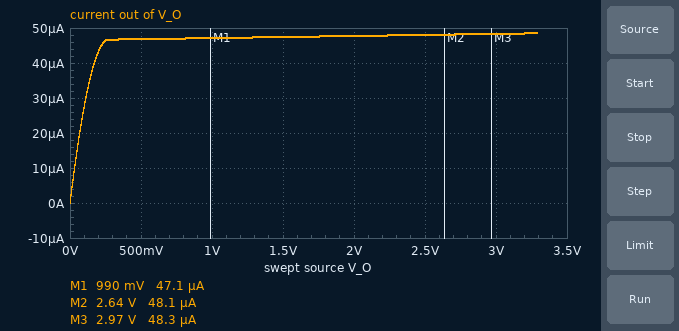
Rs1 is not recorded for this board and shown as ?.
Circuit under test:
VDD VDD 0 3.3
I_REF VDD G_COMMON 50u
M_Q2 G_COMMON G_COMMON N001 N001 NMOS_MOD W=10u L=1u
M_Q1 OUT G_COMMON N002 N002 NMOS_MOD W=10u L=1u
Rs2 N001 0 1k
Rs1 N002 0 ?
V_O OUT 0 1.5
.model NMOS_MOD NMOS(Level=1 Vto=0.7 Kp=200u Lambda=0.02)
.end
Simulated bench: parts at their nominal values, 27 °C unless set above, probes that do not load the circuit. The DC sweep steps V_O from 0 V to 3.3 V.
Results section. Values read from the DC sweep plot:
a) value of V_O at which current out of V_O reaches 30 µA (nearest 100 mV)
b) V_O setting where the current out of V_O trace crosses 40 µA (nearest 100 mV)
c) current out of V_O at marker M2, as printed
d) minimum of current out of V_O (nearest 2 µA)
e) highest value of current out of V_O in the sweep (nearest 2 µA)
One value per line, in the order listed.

100 mV
200 mV
48.1 µA
0 A
48 µA
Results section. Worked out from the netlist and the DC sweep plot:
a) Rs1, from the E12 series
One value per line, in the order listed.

1.2 kΩ
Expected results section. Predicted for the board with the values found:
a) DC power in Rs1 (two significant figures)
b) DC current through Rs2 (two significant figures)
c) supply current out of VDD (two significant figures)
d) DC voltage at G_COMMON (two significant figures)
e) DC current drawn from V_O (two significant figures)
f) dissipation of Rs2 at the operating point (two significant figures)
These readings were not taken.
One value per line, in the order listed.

2.7 µW
50 µA
50 µA
970 mV
47 µA
2.5 µW
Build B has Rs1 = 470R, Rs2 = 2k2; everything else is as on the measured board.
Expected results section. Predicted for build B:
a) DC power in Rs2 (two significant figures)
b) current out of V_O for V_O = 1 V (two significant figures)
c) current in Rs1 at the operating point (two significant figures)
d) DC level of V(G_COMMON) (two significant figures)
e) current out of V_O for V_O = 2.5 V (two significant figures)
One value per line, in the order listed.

5.5 µW
86 µA
87 µA
1.0 V
88 µA
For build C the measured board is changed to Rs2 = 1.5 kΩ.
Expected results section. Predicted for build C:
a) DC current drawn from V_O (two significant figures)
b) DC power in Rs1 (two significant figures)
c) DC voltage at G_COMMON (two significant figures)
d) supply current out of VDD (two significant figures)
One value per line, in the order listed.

55 µA
3.6 µW
1.0 V
50 µA
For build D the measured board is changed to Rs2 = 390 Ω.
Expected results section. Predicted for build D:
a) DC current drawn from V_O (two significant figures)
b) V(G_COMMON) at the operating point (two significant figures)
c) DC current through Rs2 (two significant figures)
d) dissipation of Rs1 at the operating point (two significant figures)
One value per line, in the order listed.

39 µA
940 mV
50 µA
1.8 µW
